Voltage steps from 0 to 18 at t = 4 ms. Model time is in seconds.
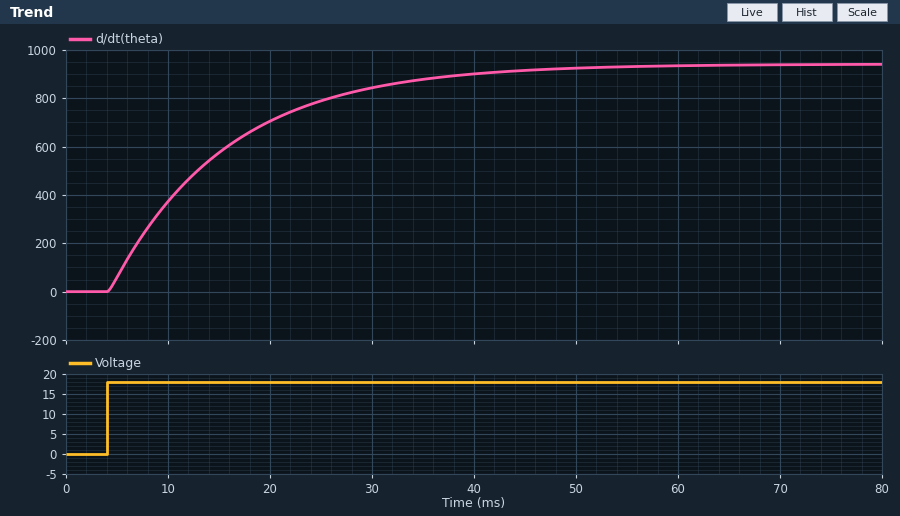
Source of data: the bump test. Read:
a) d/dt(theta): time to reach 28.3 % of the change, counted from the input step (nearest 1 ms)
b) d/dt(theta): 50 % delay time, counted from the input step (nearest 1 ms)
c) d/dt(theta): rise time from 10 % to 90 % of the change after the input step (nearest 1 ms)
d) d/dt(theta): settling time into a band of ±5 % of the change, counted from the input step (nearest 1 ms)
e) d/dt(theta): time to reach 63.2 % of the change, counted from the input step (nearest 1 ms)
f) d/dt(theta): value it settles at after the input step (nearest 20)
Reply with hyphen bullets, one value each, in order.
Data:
- 4 ms
- 8 ms
- 25 ms
- 34 ms
- 12 ms
- 940
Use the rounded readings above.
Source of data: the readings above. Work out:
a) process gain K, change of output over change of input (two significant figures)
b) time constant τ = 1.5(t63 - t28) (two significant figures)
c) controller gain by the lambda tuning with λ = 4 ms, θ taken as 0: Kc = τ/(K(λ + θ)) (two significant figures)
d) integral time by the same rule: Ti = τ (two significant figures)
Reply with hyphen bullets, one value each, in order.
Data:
- 52
- 12 ms
- 0.058
- 12 ms
